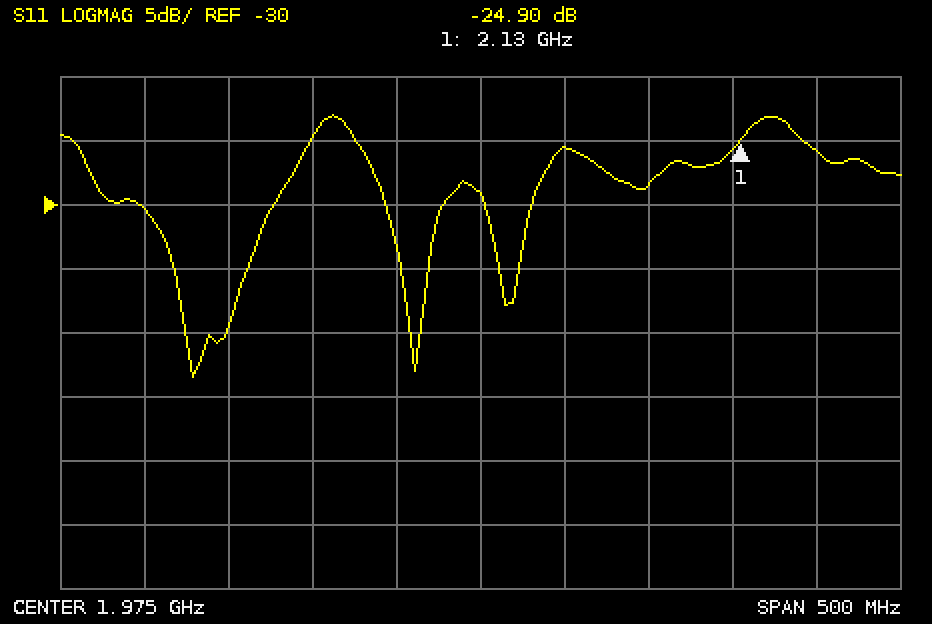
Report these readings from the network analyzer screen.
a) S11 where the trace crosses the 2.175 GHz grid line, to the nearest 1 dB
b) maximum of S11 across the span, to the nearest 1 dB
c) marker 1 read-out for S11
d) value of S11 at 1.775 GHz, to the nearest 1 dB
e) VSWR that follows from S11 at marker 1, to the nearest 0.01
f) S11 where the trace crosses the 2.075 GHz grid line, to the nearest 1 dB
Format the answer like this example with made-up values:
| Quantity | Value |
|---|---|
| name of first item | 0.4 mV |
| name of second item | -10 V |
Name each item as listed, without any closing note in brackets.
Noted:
| Quantity | Value |
|---|---|
| S11 where the trace crosses the 2.175 GHz grid line, to the nearest 1 dB | -26 dB |
| maximum of S11 across the span, to the nearest 1 dB | -23 dB |
| marker 1 read-out for S11 | -24.90 dB |
| value of S11 at 1.775 GHz, to the nearest 1 dB | -30 dB |
| VSWR that follows from S11 at marker 1, to the nearest 0.01 | 1.12 |
| S11 where the trace crosses the 2.075 GHz grid line, to the nearest 1 dB | -28 dB |
